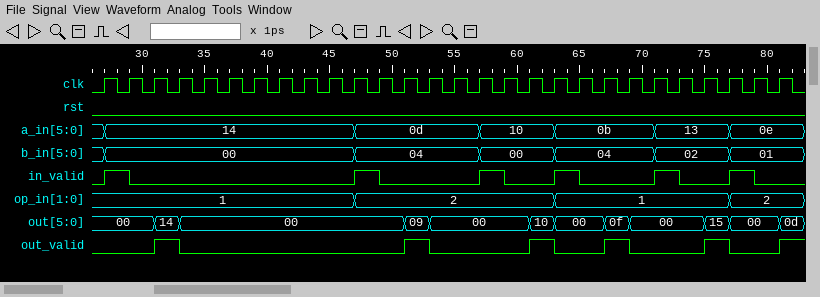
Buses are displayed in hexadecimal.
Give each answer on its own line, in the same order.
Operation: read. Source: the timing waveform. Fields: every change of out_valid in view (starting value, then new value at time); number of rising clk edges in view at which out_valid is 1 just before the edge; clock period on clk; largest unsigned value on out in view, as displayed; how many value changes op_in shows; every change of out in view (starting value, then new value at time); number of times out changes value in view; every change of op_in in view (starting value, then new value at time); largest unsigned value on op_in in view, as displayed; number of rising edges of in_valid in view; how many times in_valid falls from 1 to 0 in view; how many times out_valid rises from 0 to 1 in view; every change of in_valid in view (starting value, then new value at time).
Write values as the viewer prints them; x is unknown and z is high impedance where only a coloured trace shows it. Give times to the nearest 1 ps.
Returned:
0, 1 at 31 ps, 0 at 33 ps, 1 at 51 ps, 0 at 53 ps, 1 at 61 ps, 0 at 63 ps, 1 at 67 ps, 0 at 69 ps, 1 at 75 ps, 0 at 77 ps, 1 at 81 ps
5
2 ps
15
3
00, 14 at 31 ps, 00 at 33 ps, 09 at 51 ps, 00 at 53 ps, 10 at 61 ps, 00 at 63 ps, 0f at 67 ps, 00 at 69 ps, 15 at 75 ps, 00 at 77 ps, 0d at 81 ps
11
1, 2 at 47 ps, 1 at 63 ps, 2 at 77 ps
2
6
6
6
0, 1 at 27 ps, 0 at 29 ps, 1 at 47 ps, 0 at 49 ps, 1 at 57 ps, 0 at 59 ps, 1 at 63 ps, 0 at 65 ps, 1 at 71 ps, 0 at 73 ps, 1 at 77 ps, 0 at 79 ps
